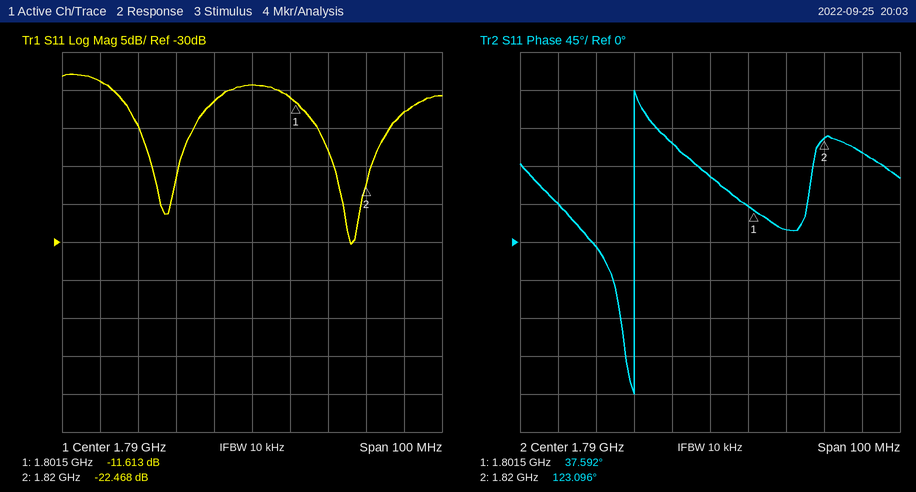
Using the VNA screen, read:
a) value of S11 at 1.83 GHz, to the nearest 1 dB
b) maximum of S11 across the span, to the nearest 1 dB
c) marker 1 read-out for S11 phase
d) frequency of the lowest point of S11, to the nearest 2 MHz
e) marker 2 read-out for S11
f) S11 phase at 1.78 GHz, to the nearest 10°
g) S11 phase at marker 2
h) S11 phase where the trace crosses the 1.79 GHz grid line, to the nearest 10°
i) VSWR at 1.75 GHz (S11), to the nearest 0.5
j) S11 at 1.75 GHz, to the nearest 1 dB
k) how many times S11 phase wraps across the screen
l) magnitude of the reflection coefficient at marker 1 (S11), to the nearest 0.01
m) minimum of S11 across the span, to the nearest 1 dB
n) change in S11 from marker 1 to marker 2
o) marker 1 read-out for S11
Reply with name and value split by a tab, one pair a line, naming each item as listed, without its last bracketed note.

value of S11 at 1.83 GHz, to the nearest 1 dB	-13 dB
maximum of S11 across the span, to the nearest 1 dB	-8 dB
marker 1 read-out for S11 phase	37.592°
frequency of the lowest point of S11, to the nearest 2 MHz	1.816 GHz
marker 2 read-out for S11	-22.468 dB
S11 phase at 1.78 GHz, to the nearest 10°	120°
S11 phase at marker 2	123.096°
S11 phase where the trace crosses the 1.79 GHz grid line, to the nearest 10°	80°
VSWR at 1.75 GHz (S11), to the nearest 0.5	2.0
S11 at 1.75 GHz, to the nearest 1 dB	-9 dB
how many times S11 phase wraps across the screen	1
magnitude of the reflection coefficient at marker 1 (S11), to the nearest 0.01	0.26
minimum of S11 across the span, to the nearest 1 dB	-30 dB
change in S11 from marker 1 to marker 2	-10.855 dB
marker 1 read-out for S11	-11.613 dB
